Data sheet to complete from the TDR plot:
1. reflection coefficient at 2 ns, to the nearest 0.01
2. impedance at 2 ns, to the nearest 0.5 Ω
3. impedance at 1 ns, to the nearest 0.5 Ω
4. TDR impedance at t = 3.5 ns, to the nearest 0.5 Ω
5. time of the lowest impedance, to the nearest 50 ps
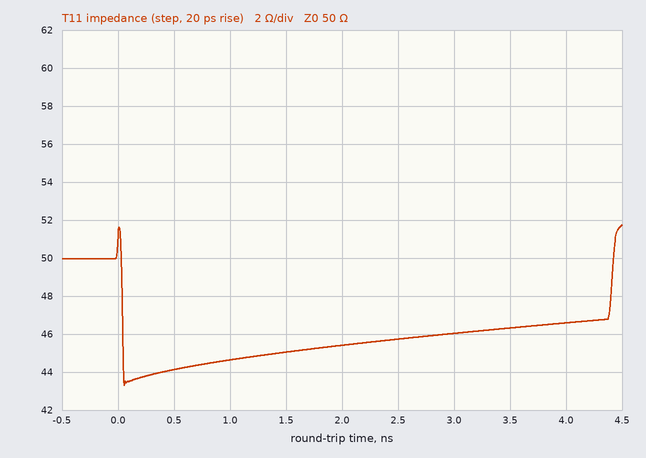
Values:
-0.05
45.5 Ω
44.5 Ω
46.5 Ω
50 ps
